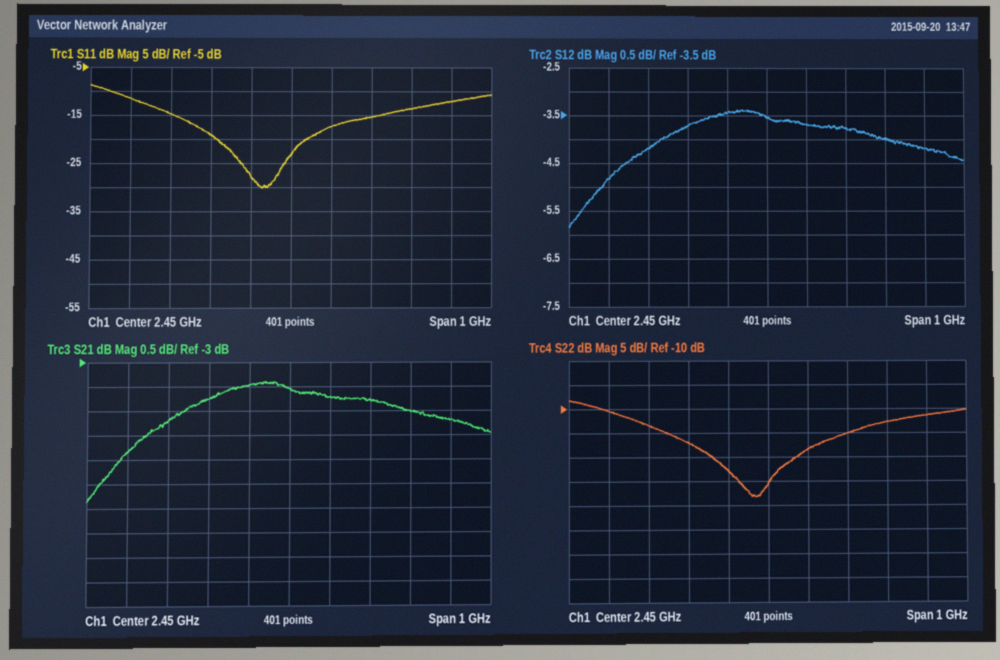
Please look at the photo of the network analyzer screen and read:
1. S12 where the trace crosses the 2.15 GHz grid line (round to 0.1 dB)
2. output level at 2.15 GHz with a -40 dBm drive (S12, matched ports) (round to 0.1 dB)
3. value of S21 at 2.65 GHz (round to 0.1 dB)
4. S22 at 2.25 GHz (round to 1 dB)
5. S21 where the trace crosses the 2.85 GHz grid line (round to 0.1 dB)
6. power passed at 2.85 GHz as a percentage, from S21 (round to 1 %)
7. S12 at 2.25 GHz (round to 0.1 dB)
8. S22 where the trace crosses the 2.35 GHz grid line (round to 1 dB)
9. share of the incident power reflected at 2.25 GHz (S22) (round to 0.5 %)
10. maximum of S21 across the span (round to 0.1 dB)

-4.2 dB
-44.2 dBm
-3.8 dB
-17 dB
-4.2 dB
38 %
-3.7 dB
-23 dB
2.0 %
-3.4 dB
